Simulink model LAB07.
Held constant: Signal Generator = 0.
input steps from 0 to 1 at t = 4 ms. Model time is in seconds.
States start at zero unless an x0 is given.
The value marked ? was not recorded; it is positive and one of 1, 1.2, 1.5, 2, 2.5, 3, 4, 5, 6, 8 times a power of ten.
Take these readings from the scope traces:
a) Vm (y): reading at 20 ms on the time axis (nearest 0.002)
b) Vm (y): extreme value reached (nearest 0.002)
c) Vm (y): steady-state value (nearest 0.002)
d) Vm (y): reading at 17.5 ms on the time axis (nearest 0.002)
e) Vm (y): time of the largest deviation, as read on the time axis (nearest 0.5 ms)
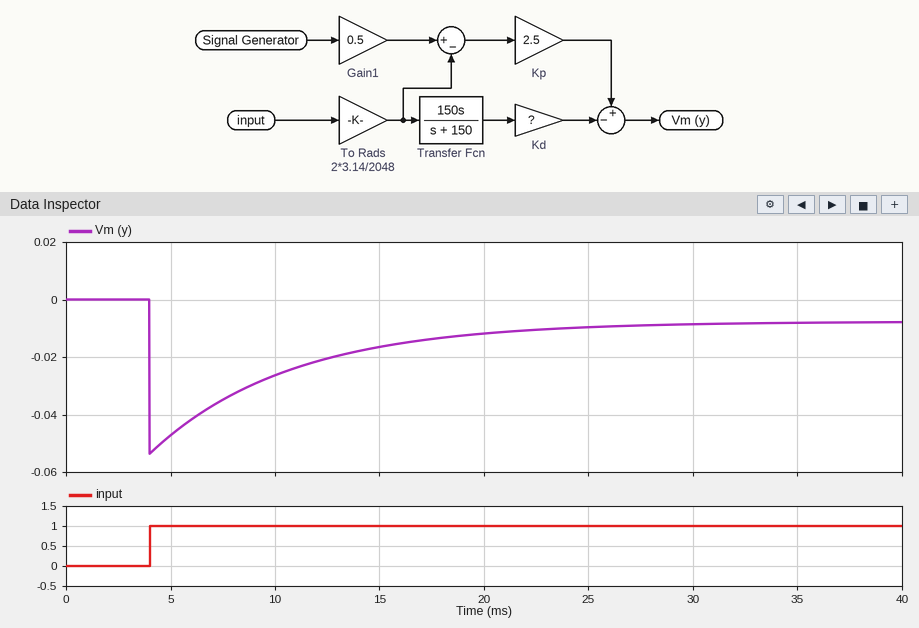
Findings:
-0.012
-0.054
-0.008
-0.014
4.0 ms
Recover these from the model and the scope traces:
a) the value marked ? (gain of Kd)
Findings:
0.1
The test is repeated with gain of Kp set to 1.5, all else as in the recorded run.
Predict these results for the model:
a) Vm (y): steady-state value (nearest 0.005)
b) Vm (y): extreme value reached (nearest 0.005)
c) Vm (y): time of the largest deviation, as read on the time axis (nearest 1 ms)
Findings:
-0.005
-0.050
4 ms
